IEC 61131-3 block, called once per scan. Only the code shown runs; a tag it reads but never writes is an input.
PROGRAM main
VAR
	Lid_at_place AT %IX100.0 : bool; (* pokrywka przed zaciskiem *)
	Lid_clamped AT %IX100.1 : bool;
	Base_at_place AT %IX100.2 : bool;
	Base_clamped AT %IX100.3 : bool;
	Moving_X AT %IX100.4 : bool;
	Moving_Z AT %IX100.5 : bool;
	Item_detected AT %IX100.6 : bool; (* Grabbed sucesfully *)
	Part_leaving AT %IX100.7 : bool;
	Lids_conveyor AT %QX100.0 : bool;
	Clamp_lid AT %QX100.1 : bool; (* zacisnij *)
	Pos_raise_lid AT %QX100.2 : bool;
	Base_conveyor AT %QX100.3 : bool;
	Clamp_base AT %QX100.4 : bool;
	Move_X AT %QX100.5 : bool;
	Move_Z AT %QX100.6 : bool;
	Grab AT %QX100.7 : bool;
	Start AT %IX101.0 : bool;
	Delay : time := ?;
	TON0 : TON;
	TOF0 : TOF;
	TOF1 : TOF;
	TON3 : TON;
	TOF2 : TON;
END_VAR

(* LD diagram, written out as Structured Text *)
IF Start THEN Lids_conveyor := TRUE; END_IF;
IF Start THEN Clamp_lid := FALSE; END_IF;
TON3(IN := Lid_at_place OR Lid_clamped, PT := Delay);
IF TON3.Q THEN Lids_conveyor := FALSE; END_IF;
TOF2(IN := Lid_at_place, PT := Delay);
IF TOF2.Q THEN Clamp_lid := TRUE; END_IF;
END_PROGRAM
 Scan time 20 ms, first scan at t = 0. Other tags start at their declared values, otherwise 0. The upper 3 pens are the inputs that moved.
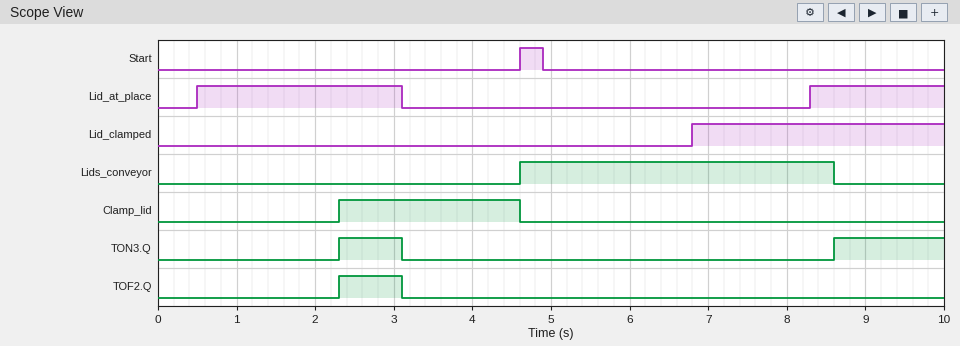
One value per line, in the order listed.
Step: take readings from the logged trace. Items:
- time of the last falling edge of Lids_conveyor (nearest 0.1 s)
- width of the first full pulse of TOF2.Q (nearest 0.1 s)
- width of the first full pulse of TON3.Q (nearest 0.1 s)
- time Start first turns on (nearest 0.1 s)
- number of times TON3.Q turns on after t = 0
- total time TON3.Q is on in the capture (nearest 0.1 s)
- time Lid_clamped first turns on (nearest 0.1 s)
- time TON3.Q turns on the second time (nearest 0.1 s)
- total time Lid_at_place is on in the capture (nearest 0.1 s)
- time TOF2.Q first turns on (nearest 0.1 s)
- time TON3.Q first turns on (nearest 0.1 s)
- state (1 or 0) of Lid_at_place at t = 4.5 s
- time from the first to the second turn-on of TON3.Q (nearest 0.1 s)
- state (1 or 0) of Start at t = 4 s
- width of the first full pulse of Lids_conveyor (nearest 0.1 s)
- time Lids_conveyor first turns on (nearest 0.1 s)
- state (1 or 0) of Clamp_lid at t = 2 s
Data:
8.6 s
0.8 s
0.8 s
4.6 s
2
2.2 s
6.8 s
8.6 s
4.3 s
2.3 s
2.3 s
0
6.3 s
0
4.0 s
4.6 s
0
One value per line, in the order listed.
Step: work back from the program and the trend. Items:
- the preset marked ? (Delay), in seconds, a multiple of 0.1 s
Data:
1.8 s
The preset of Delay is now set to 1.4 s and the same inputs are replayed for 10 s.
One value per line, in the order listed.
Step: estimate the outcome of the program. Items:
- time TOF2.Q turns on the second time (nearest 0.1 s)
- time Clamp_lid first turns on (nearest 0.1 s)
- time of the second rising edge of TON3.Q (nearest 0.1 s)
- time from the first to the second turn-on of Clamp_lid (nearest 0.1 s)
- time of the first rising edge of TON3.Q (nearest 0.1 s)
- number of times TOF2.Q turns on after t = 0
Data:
9.7 s
1.9 s
8.2 s
7.8 s
1.9 s
2
